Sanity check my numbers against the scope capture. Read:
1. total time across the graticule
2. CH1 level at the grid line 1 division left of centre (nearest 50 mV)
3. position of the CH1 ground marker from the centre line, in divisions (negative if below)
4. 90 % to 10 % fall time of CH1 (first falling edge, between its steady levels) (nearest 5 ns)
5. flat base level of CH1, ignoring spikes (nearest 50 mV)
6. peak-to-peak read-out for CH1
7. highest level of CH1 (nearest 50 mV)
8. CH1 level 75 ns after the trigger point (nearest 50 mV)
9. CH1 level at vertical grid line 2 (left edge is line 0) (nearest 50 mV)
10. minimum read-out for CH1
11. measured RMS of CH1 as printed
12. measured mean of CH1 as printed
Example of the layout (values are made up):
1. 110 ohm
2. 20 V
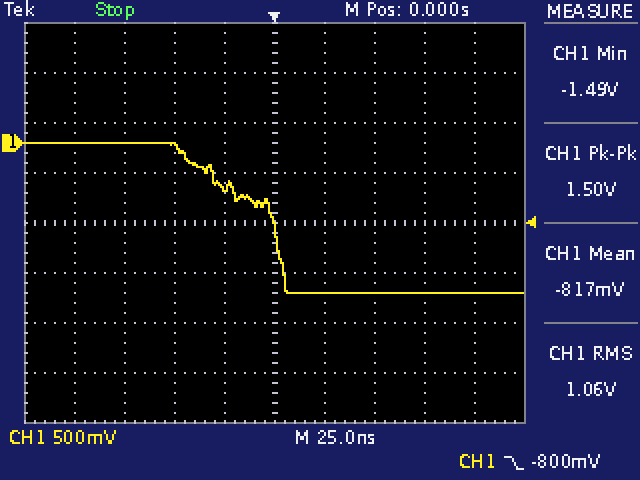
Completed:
1. 250 ns
2. -450 mV
3. +1.6 div
4. 50 ns
5. -1.50 V
6. 1.50 V
7. 0 mV
8. -1.50 V
9. 0 mV
10. -1.49 V
11. 1.06 V
12. -817 mV
